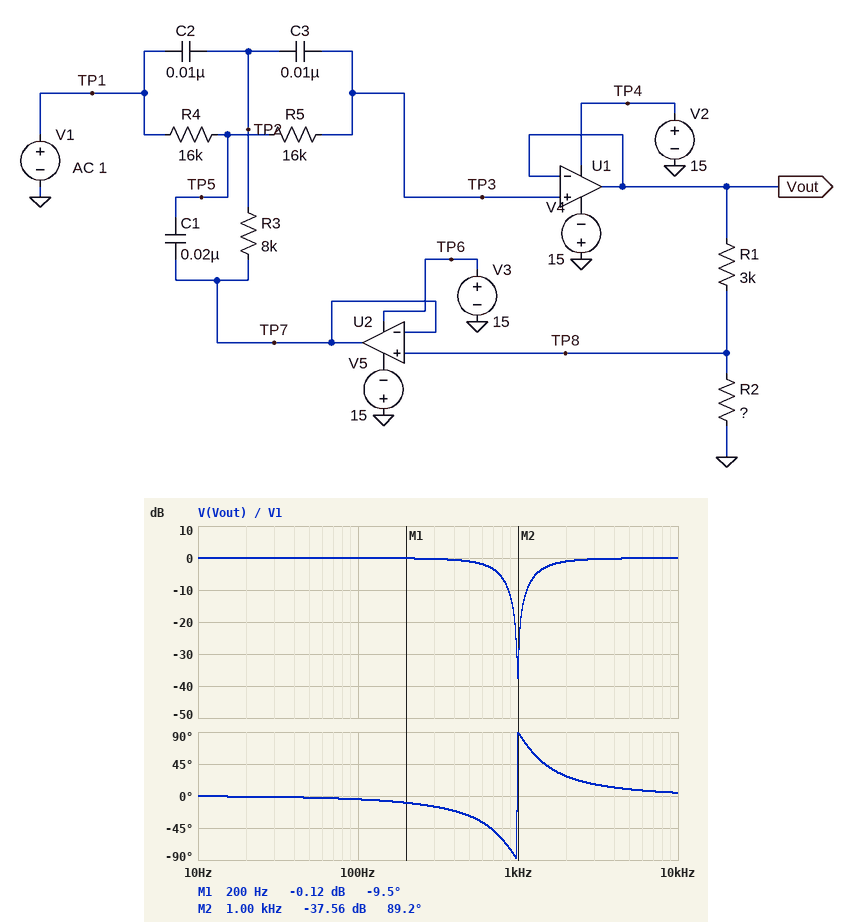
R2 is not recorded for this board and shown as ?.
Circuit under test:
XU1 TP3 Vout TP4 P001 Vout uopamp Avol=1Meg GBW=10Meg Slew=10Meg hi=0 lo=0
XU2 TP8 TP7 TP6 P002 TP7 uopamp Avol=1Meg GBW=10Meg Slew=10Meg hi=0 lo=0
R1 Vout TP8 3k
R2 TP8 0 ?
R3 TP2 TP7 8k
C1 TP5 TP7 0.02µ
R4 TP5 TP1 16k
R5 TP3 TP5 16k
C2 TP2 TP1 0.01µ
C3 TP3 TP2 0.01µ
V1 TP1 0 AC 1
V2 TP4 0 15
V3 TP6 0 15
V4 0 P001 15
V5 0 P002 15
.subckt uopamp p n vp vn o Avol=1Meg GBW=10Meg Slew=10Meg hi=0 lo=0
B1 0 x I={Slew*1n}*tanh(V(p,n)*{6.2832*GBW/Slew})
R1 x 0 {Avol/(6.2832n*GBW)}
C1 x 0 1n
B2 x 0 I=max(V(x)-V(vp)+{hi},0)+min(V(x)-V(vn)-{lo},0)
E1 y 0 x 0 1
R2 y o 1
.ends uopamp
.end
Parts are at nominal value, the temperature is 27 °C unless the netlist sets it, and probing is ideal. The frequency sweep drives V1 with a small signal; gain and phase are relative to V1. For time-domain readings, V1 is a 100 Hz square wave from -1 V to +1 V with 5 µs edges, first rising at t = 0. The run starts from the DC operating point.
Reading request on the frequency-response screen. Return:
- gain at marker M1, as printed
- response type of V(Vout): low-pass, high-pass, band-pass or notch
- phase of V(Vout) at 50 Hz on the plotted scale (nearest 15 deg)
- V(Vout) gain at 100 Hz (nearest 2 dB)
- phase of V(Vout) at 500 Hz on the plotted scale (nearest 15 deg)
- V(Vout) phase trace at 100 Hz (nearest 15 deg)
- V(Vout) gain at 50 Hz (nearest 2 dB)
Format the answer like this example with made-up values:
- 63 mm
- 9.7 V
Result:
- -0.12 dB
- notch
- 0 deg
- 0 dB
- -30 deg
- 0 deg
- 0 dB
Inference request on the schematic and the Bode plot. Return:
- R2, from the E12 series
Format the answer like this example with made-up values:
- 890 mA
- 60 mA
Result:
- 12 kΩ
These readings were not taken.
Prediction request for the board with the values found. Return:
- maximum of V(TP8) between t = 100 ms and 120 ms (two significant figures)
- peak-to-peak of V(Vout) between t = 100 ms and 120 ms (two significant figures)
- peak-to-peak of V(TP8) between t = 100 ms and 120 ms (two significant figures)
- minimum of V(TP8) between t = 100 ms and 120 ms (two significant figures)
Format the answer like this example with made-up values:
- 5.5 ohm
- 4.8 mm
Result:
- 1.0 V
- 2.5 V
- 2.0 V
- -1.0 V
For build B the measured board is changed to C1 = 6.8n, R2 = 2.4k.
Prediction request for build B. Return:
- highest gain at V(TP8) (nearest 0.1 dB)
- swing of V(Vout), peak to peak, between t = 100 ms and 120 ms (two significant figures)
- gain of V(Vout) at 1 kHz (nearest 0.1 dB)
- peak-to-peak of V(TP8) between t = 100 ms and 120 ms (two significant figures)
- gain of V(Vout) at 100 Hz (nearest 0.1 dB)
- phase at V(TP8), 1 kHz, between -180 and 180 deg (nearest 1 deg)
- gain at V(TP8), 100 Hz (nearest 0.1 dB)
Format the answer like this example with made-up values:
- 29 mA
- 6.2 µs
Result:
- -7.0 dB
- 2.0 V
- -10.8 dB
- 890 mV
- -0.2 dB
- -19 deg
- -7.2 dB
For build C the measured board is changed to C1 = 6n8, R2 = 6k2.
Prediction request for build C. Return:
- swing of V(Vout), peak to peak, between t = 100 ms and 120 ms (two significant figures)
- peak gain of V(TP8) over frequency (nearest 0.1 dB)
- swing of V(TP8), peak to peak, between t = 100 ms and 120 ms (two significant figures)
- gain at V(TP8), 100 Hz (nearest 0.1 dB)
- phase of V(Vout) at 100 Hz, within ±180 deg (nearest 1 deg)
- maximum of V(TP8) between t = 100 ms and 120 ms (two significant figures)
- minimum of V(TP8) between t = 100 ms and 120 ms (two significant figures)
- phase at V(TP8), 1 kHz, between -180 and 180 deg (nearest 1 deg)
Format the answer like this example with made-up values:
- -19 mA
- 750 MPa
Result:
- 2.0 V
- -3.4 dB
- 1.4 V
- -3.5 dB
- -5 deg
- 680 mV
- -680 mV
- -16 deg
